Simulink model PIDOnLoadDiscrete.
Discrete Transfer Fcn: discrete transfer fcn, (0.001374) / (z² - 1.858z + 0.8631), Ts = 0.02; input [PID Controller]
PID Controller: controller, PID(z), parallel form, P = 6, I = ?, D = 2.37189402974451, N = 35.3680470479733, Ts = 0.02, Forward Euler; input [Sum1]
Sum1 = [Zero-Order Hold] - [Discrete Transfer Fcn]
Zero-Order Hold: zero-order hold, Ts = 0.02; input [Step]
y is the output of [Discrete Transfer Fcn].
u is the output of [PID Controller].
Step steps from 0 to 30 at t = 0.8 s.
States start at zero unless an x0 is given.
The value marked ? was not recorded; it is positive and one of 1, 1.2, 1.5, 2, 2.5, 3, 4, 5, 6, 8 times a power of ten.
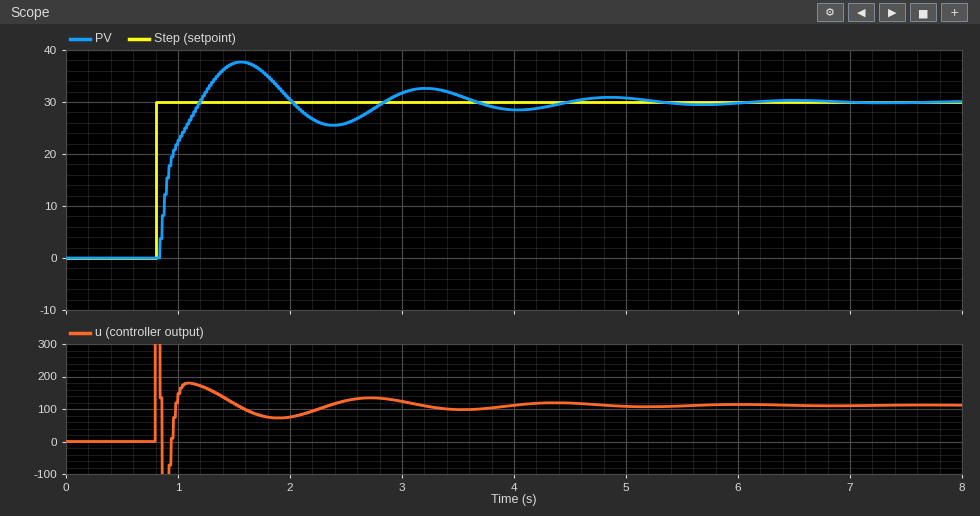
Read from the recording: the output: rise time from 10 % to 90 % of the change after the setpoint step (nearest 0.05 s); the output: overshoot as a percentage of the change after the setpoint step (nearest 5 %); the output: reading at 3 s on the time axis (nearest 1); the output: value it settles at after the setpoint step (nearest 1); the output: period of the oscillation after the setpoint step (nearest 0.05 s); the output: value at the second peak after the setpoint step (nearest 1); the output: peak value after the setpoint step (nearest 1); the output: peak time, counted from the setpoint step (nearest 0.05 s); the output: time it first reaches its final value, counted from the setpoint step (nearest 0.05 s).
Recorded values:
0.30 s
25 %
32
30
1.65 s
33
38
0.75 s
0.40 s
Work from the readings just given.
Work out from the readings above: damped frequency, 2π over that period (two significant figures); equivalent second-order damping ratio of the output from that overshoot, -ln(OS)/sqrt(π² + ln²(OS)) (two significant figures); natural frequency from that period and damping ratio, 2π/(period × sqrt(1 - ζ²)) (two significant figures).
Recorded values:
3.8 rad/s
0.40
4.2 rad/s
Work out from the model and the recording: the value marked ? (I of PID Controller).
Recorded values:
60
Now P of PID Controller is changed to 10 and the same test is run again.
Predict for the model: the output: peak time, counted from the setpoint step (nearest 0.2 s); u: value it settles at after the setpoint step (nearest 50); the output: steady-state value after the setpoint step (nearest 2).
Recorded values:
0.6 s
100
30
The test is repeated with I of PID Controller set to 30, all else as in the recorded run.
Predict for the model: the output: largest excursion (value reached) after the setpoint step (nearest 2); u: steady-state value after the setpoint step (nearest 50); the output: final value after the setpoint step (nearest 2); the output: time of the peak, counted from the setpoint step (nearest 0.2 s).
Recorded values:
34
100
30
1.2 s
